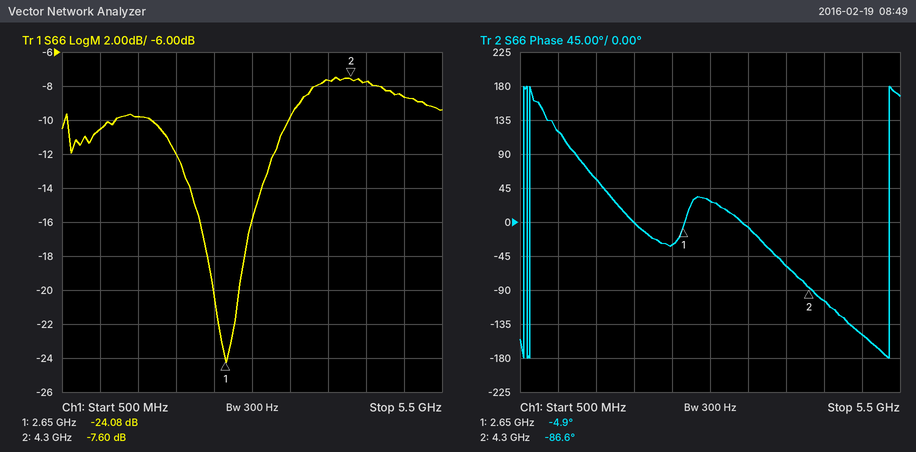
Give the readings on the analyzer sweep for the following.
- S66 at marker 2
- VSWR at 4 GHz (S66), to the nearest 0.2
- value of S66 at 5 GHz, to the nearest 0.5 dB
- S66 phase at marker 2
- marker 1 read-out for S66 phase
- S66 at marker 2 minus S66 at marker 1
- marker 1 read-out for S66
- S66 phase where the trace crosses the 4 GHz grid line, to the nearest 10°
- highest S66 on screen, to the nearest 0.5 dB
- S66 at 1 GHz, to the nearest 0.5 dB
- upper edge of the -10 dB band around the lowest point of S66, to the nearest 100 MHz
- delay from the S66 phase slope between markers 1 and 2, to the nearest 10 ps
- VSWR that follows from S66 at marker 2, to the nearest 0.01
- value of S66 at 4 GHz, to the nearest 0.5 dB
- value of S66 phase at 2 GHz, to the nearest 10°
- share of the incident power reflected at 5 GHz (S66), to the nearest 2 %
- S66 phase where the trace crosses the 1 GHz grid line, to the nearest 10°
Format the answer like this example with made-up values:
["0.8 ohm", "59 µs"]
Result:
["-7.60 dB", "2.4", "-8.5 dB", "-86.6°", "-4.9°", "16.48 dB", "-24.08 dB", "-60°", "-7.5 dB", "-10.5 dB", "3.5 GHz", "140 ps", "2.43", "-7.5 dB", "0°", "14 %", "120°"]
